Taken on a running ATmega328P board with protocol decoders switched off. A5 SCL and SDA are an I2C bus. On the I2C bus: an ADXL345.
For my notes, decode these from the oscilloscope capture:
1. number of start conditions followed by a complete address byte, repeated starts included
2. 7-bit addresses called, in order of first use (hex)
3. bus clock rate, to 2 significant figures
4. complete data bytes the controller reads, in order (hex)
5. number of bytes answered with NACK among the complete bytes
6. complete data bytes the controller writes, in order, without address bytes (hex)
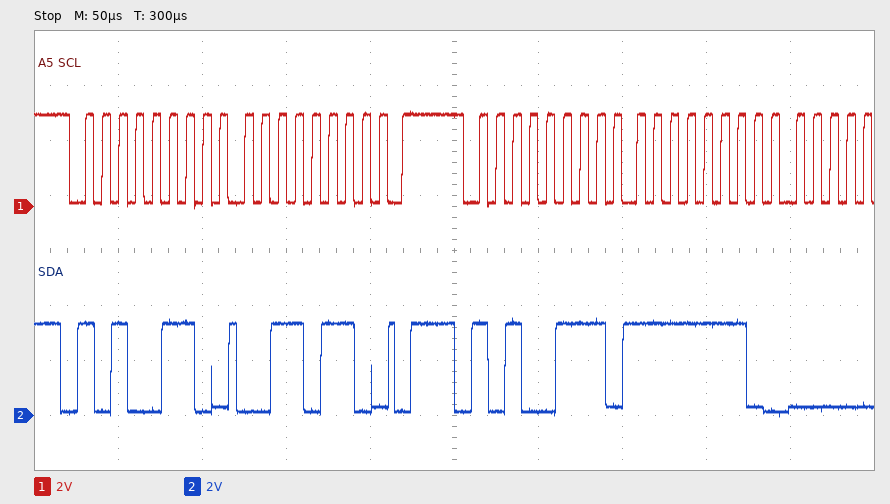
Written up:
2
0x53
100 kHz
FE
0
36
